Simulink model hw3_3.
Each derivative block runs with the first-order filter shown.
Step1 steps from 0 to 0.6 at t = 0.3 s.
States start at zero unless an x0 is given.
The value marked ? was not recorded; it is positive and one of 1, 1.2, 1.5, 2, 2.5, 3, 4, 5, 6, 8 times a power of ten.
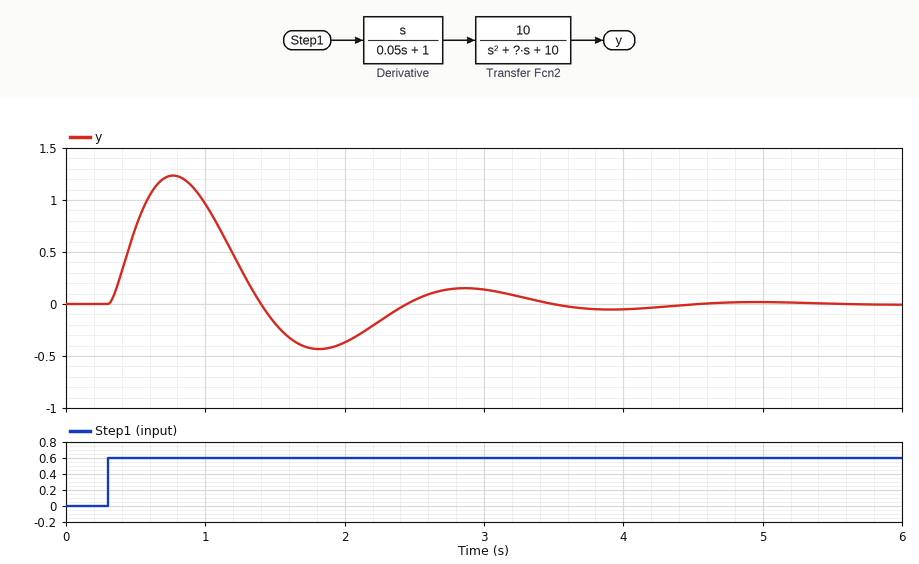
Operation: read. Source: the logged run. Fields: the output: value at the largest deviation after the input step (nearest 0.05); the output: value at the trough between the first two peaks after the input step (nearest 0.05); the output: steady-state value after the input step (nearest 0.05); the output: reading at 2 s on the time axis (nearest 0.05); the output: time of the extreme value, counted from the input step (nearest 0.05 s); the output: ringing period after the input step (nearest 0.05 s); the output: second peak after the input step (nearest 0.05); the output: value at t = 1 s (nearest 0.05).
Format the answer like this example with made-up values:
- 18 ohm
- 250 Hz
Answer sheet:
- 1.25
- -0.45
- 0.00
- -0.35
- 0.45 s
- 2.10 s
- 0.15
- 0.95
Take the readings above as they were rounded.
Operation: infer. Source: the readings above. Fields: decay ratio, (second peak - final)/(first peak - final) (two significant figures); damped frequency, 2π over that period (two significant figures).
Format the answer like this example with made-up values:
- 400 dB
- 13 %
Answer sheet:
- 0.12
- 3.0 rad/s
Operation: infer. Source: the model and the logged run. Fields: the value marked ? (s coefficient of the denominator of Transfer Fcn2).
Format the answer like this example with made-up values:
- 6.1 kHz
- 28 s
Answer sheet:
- 2
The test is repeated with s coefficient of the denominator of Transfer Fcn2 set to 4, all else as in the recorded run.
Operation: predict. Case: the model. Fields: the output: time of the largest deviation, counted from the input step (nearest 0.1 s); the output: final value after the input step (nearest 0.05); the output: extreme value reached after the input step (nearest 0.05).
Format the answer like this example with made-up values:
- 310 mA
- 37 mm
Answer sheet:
- 0.4 s
- 0.00
- 0.90
